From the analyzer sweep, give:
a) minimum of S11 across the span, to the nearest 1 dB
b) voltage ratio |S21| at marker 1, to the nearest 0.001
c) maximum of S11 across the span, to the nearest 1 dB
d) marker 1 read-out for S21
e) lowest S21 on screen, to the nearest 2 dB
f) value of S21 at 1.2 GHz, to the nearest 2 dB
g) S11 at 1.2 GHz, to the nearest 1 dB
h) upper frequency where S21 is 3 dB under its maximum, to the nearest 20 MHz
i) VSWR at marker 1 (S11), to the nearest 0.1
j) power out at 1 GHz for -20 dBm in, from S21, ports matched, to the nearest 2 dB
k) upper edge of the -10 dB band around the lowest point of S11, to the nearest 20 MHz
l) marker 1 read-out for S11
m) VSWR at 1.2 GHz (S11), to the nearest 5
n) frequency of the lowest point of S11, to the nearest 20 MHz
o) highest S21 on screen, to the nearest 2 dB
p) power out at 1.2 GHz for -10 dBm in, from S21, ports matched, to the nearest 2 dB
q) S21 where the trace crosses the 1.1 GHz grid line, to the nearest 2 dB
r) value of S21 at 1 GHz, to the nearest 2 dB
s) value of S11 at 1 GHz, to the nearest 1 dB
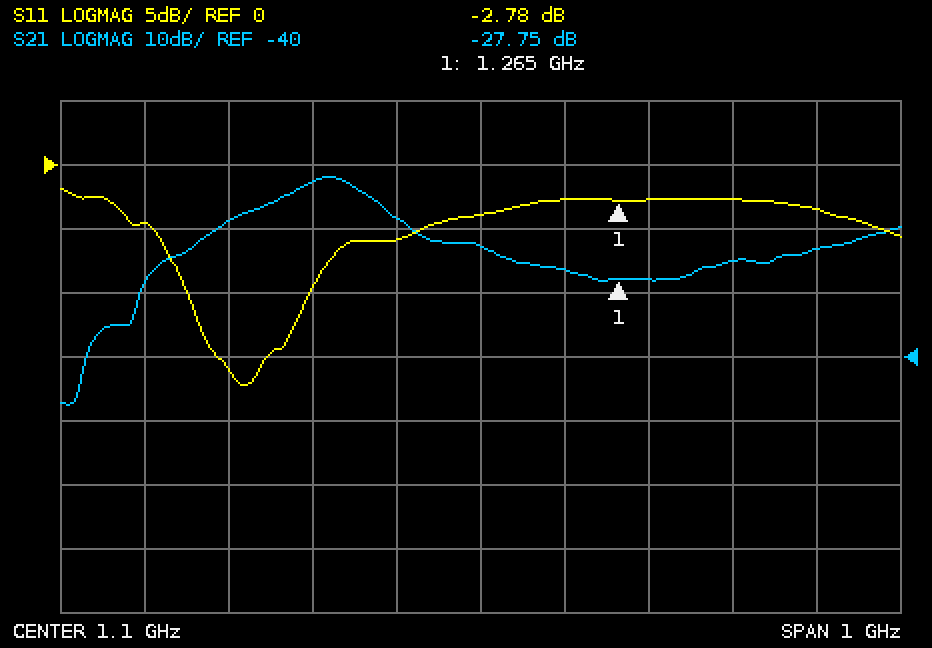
-17 dB
0.041
-2 dB
-27.75 dB
-48 dB
-26 dB
-3 dB
960 MHz
6.3
-38 dBm
900 MHz
-2.78 dB
5
820 MHz
-12 dB
-36 dBm
-22 dB
-18 dB
-6 dB
